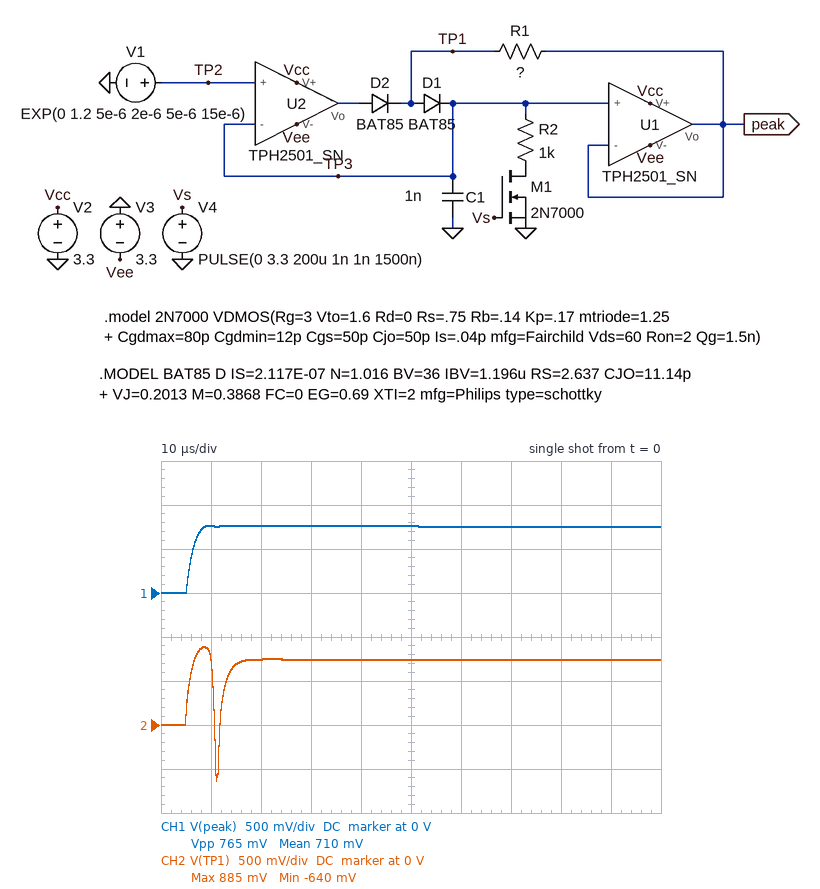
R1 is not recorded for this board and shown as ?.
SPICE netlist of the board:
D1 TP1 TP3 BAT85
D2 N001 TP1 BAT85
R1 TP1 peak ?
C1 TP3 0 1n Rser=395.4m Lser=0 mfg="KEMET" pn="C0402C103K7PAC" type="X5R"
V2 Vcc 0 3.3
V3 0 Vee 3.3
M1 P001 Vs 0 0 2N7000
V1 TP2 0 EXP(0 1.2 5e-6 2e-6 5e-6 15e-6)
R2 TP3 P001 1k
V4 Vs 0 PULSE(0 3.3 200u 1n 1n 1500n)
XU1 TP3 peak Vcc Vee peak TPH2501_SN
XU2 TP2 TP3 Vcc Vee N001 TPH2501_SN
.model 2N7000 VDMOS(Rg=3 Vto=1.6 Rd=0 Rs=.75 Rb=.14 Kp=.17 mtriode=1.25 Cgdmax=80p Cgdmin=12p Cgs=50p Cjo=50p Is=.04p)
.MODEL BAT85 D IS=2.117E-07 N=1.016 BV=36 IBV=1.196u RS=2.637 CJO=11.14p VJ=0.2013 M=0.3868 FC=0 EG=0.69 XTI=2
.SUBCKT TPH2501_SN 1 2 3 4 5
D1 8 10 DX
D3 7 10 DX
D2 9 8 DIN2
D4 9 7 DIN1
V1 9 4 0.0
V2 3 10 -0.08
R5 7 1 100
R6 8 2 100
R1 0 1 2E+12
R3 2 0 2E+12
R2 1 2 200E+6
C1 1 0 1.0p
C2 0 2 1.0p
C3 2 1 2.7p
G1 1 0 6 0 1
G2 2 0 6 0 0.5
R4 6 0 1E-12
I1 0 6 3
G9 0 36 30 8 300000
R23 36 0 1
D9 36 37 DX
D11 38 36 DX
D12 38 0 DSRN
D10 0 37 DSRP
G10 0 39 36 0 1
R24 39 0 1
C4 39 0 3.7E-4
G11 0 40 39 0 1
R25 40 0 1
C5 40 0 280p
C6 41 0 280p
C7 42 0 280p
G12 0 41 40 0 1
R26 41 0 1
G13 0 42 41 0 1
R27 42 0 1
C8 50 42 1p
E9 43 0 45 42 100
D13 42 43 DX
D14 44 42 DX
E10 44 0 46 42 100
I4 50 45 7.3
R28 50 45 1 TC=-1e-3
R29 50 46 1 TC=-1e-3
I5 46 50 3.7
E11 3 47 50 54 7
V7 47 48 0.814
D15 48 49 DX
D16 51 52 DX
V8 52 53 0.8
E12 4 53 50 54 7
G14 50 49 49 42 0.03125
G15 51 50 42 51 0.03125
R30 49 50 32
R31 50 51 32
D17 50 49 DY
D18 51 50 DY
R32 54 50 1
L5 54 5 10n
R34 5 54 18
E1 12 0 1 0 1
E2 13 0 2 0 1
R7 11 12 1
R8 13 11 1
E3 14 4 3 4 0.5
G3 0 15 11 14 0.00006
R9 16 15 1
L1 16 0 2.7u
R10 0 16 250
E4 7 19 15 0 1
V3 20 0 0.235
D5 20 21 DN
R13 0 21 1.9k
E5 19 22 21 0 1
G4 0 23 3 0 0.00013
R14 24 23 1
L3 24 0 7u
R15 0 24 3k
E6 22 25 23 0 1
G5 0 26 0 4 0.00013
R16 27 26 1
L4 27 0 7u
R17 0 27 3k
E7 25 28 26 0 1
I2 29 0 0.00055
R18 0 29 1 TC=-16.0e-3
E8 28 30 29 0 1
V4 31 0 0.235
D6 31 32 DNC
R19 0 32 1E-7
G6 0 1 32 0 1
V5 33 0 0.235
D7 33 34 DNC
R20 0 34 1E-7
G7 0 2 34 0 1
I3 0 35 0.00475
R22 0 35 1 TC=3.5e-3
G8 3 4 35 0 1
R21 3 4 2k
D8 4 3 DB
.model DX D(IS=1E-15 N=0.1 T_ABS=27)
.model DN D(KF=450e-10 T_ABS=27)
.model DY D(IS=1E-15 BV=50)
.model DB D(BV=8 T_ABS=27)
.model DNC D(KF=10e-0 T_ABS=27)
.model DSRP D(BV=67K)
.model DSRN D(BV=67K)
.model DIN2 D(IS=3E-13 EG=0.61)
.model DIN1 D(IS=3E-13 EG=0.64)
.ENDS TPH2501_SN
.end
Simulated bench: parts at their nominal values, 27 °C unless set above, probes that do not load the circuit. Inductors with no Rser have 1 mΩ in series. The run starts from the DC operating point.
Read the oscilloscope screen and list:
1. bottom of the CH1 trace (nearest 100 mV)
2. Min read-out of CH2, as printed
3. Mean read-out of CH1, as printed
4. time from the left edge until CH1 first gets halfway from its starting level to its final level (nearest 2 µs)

0 V
-640 mV
710 mV
6 µs
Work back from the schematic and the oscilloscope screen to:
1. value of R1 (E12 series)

120 kΩ
